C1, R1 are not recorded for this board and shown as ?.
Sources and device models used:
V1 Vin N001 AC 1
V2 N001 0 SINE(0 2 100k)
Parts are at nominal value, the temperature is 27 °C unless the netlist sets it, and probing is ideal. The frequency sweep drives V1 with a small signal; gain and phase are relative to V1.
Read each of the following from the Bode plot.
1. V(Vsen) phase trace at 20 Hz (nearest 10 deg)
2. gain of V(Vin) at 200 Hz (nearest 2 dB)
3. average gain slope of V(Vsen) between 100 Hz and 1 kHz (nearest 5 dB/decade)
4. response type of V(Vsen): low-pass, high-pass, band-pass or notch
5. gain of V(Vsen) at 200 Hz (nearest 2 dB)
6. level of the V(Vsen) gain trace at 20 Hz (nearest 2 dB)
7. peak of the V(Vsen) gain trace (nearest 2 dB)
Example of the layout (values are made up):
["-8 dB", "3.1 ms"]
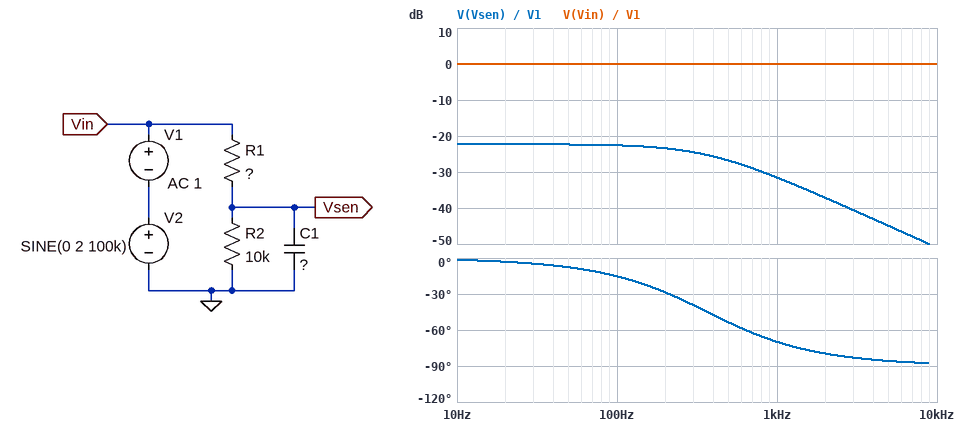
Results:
["0 deg", "0 dB", "-10 dB/decade", "low-pass", "-24 dB", "-22 dB", "-22 dB"]
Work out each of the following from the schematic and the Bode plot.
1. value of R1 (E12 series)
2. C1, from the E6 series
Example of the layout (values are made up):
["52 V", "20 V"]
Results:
["120 kΩ", "47 nF"]
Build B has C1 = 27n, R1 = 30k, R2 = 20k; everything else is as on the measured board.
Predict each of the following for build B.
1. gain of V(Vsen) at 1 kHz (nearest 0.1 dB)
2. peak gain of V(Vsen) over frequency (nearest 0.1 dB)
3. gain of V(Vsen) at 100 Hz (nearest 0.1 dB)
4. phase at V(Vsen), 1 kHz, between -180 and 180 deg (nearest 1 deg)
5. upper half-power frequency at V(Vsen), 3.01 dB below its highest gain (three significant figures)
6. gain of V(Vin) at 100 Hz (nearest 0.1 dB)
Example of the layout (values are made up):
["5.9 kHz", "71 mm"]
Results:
["-15.1 dB", "-8.0 dB", "-8.1 dB", "-64 deg", "491 Hz", "0 dB"]
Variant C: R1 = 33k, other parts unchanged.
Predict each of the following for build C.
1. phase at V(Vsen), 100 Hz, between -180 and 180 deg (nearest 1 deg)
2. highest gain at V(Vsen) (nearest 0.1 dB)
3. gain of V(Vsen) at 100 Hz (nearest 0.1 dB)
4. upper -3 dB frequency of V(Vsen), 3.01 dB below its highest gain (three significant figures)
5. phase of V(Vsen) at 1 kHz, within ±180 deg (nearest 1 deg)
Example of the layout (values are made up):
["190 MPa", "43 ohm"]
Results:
["-13 deg", "-12.7 dB", "-12.9 dB", "441 Hz", "-66 deg"]
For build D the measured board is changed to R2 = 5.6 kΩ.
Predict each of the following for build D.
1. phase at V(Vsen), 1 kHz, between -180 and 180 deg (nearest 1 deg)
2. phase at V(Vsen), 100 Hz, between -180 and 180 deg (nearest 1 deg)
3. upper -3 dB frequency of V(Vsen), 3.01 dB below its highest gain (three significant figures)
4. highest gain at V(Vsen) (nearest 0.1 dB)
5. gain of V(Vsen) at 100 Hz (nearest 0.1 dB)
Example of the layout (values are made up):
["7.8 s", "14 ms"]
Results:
["-58 deg", "-9 deg", "633 Hz", "-27.0 dB", "-27.1 dB"]
